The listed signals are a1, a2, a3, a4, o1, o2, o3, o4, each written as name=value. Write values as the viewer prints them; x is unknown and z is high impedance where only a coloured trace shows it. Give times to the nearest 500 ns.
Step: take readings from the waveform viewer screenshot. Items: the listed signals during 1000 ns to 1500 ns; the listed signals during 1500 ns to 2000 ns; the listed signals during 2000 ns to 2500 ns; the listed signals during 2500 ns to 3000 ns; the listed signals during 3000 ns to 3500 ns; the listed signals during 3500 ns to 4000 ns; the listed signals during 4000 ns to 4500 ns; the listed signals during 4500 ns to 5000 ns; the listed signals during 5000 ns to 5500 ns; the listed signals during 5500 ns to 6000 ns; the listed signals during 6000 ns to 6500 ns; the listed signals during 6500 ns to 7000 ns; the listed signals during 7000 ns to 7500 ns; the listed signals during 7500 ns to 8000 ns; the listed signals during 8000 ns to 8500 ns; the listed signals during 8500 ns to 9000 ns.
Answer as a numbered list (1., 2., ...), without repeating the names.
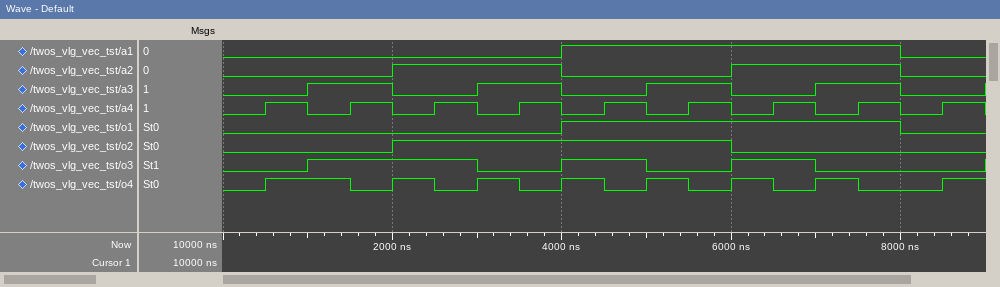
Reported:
1. a1=0, a2=0, a3=1, a4=0, o1=0, o2=0, o3=1, o4=1
2. a1=0, a2=0, a3=1, a4=1, o1=0, o2=0, o3=1, o4=0
3. a1=0, a2=1, a3=0, a4=0, o1=0, o2=1, o3=1, o4=1
4. a1=0, a2=1, a3=0, a4=1, o1=0, o2=1, o3=1, o4=0
5. a1=0, a2=1, a3=1, a4=0, o1=0, o2=1, o3=0, o4=1
6. a1=0, a2=1, a3=1, a4=1, o1=0, o2=1, o3=0, o4=0
7. a1=1, a2=0, a3=0, a4=0, o1=1, o2=1, o3=1, o4=1
8. a1=1, a2=0, a3=0, a4=1, o1=1, o2=1, o3=1, o4=0
9. a1=1, a2=0, a3=1, a4=0, o1=1, o2=1, o3=0, o4=1
10. a1=1, a2=0, a3=1, a4=1, o1=1, o2=1, o3=0, o4=0
11. a1=1, a2=1, a3=0, a4=0, o1=1, o2=0, o3=1, o4=1
12. a1=1, a2=1, a3=0, a4=1, o1=1, o2=0, o3=1, o4=0
13. a1=1, a2=1, a3=1, a4=0, o1=1, o2=0, o3=0, o4=1
14. a1=1, a2=1, a3=1, a4=1, o1=1, o2=0, o3=0, o4=0
15. a1=0, a2=0, a3=0, a4=0, o1=0, o2=0, o3=0, o4=0
16. a1=0, a2=0, a3=0, a4=1, o1=0, o2=0, o3=0, o4=1
